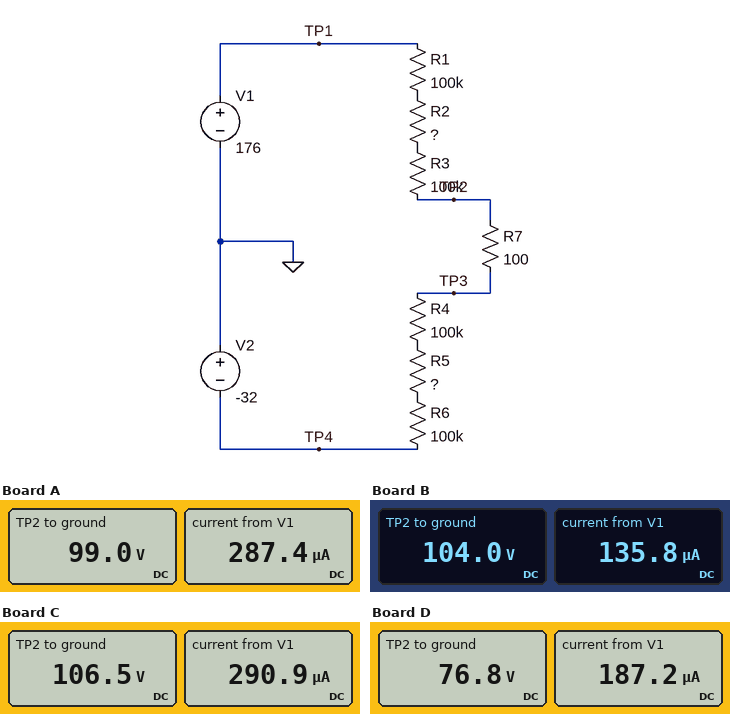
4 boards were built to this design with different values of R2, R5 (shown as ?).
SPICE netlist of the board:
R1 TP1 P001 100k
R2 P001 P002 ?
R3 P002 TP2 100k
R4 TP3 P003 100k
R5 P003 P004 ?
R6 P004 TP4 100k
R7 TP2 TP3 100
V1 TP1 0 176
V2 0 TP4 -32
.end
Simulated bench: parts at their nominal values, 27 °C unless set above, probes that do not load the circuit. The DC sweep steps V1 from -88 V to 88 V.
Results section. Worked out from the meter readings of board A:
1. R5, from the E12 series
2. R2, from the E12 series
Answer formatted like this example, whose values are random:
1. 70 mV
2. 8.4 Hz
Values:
1. 33 kΩ
2. 68 kΩ
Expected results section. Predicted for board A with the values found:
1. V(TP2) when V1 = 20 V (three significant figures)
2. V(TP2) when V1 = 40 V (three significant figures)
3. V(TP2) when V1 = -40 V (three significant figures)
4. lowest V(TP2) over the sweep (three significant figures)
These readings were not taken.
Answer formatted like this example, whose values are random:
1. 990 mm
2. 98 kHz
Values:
1. 26.4 V
2. 35.7 V
3. -1.49 V
4. -23.8 V
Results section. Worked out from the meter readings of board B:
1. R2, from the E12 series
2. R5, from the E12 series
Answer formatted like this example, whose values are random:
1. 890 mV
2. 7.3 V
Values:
1. 330 kΩ
2. 330 kΩ
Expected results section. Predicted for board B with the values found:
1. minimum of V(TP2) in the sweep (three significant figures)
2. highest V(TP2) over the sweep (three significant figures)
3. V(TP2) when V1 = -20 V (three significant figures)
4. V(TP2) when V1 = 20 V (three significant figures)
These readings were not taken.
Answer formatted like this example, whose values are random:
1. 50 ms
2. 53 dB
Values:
1. -28.0 V
2. 60.0 V
3. 6.00 V
4. 26.0 V
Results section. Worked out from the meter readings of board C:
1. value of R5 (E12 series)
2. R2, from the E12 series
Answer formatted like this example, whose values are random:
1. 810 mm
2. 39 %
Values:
1. 56 kΩ
2. 39 kΩ
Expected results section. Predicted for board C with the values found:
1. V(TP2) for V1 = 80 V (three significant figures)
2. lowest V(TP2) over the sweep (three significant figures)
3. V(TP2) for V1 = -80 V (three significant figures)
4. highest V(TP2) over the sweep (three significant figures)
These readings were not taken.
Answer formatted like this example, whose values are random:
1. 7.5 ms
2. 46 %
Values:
1. 56.8 V
2. -30.1 V
3. -25.9 V
4. 61.0 V
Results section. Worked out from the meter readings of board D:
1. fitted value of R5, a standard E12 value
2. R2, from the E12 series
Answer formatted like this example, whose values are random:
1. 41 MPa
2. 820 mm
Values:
1. 39 kΩ
2. 330 kΩ
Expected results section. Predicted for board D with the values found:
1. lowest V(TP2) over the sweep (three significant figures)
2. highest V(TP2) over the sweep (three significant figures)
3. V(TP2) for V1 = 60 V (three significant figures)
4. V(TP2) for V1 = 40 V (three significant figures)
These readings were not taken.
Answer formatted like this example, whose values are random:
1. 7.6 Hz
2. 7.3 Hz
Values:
1. -5.31 V
2. 49.4 V
3. 40.7 V
4. 34.5 V
